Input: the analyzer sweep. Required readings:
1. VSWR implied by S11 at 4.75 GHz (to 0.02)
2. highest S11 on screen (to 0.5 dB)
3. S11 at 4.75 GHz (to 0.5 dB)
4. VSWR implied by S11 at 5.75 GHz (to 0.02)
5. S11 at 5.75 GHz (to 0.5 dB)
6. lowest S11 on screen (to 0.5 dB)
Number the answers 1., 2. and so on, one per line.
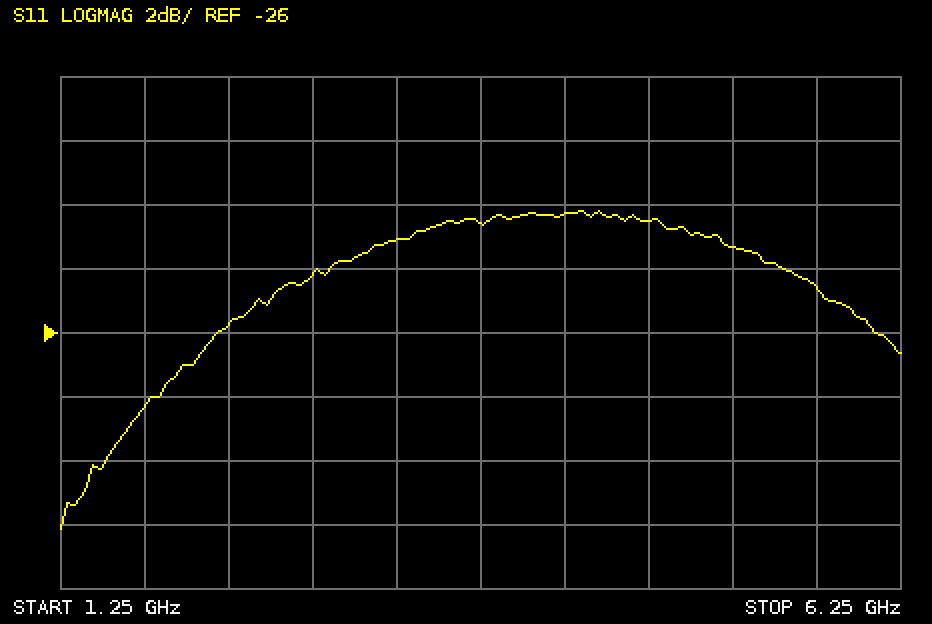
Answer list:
1. 1.16
2. -22.0 dB
3. -22.5 dB
4. 1.12
5. -24.5 dB
6. -32.0 dB
